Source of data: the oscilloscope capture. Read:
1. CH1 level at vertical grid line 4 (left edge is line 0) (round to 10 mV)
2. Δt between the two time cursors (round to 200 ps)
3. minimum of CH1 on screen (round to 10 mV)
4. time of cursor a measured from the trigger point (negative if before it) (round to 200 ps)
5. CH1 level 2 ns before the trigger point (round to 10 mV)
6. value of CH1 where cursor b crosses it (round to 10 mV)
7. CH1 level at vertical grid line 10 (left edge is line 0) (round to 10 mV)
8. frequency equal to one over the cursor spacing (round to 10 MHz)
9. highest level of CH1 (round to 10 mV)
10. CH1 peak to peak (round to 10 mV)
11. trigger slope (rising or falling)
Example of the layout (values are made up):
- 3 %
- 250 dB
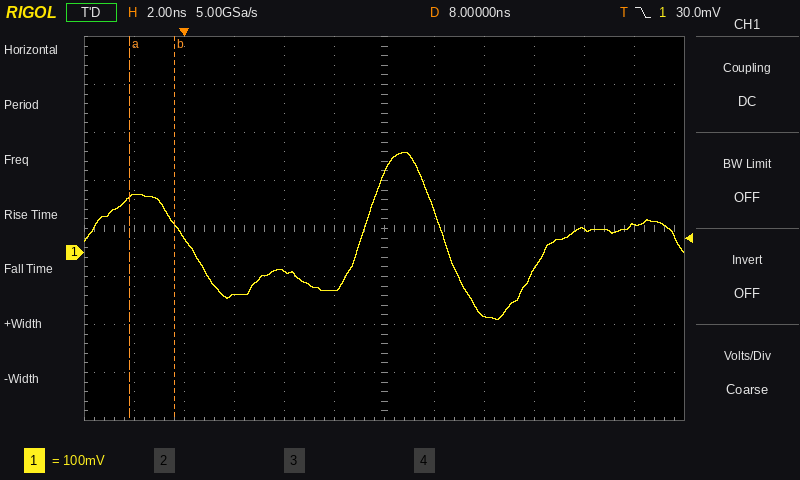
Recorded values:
- -40 mV
- 1.8 ns
- -140 mV
- -2.2 ns
- 120 mV
- 60 mV
- 50 mV
- 560 MHz
- 210 mV
- 350 mV
- falling
